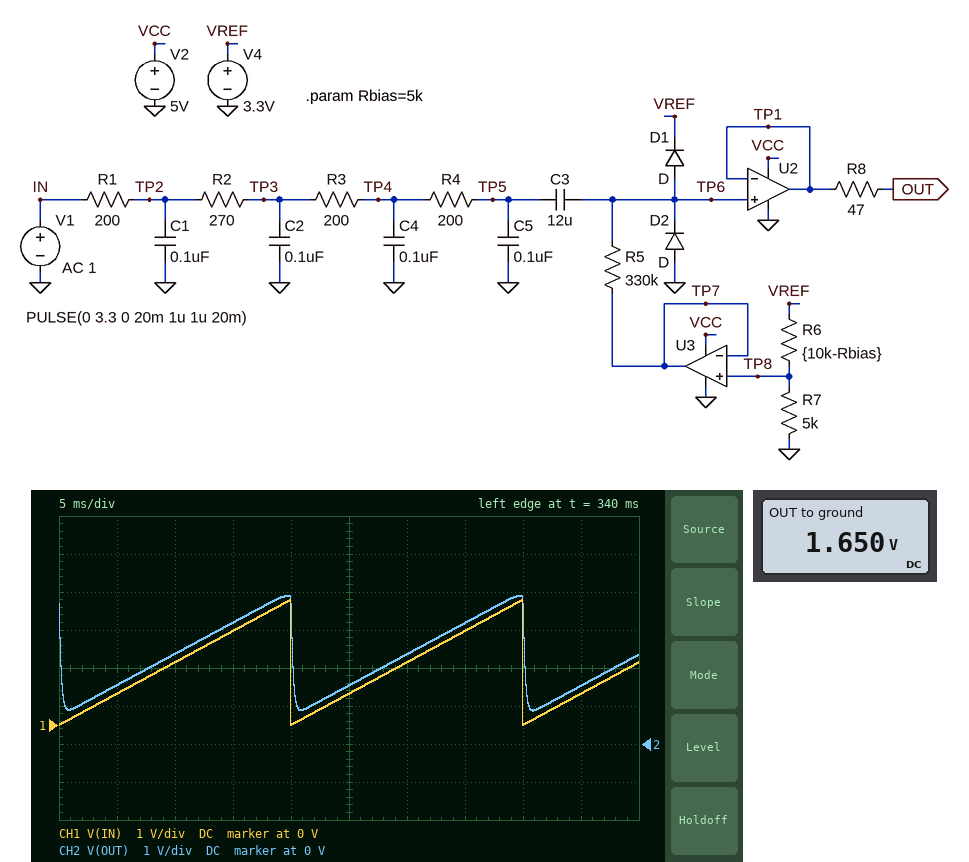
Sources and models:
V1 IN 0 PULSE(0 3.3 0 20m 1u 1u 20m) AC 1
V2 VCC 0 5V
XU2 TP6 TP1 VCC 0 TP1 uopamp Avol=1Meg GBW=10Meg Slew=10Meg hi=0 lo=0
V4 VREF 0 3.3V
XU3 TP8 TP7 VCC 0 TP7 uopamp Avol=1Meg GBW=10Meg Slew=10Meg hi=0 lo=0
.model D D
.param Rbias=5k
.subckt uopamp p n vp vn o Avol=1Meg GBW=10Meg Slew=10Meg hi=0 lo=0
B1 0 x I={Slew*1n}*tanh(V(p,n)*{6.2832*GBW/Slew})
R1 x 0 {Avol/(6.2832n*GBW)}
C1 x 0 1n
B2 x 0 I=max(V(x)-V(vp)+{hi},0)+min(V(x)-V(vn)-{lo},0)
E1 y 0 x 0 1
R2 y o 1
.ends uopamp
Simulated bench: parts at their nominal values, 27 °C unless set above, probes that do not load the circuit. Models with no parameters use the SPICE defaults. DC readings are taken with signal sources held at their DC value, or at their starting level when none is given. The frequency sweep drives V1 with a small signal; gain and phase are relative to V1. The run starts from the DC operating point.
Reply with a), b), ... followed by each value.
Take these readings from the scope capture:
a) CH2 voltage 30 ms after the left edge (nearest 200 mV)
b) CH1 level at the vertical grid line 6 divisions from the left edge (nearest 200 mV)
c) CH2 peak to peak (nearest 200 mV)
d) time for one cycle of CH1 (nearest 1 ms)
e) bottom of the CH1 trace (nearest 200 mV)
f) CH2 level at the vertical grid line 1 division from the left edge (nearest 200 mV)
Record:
a) 2.4 V
b) 1.6 V
c) 3.0 V
d) 20 ms
e) 0 V
f) 1.6 V
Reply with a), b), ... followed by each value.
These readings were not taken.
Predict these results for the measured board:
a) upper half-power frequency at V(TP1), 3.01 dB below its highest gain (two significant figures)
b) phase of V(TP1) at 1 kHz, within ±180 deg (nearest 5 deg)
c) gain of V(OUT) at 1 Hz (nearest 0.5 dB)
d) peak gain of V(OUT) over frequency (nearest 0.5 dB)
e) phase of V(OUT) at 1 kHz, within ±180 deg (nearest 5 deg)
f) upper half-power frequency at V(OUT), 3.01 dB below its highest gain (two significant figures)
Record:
a) 850 Hz
b) -60 deg
c) 0 dB
d) 0 dB
e) -60 deg
f) 850 Hz
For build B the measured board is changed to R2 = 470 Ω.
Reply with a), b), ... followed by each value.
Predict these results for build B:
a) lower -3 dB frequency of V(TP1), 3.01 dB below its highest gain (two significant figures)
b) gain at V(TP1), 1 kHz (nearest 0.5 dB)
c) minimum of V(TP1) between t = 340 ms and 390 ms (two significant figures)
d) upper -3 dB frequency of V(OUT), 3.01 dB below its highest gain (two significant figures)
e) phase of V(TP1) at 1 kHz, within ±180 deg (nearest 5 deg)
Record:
a) 40 mHz
b) -5.5 dB
c) 940 mV
d) 650 Hz
e) -70 deg
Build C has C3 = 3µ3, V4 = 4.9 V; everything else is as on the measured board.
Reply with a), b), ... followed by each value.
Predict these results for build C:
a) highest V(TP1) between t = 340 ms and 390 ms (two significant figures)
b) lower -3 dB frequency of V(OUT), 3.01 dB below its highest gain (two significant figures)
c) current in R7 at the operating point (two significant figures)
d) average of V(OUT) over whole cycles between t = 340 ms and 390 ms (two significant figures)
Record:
a) 5.0 V
b) 150 mHz
c) 490 µA
d) 3.6 V
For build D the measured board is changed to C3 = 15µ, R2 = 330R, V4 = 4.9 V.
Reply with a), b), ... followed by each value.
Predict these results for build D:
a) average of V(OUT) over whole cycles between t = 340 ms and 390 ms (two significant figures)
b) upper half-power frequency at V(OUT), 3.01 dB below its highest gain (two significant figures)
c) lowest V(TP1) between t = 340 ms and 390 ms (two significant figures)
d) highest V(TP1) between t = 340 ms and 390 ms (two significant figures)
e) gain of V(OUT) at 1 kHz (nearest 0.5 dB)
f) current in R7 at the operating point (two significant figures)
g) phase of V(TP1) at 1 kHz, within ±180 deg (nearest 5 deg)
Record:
a) 3.9 V
b) 780 Hz
c) 2.4 V
d) 5.0 V
e) -4.5 dB
f) 490 µA
g) -65 deg
